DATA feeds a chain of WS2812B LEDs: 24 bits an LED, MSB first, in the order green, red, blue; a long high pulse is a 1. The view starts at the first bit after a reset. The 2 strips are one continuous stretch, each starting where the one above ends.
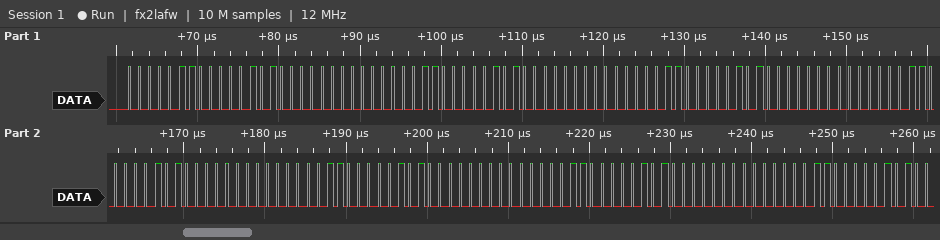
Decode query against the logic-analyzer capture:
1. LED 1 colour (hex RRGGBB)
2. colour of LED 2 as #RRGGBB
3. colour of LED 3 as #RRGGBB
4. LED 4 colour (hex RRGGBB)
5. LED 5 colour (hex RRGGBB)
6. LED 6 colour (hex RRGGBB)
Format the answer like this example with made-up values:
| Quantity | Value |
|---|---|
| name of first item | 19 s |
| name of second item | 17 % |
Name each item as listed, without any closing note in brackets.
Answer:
| Quantity | Value |
|---|---|
| LED 1 colour | #0A0600 |
| colour of LED 2 as #RRGGBB | #0A0600 |
| colour of LED 3 as #RRGGBB | #0A0600 |
| LED 4 colour | #0A0600 |
| LED 5 colour | #0A0600 |
| LED 6 colour | #0A0600 |
